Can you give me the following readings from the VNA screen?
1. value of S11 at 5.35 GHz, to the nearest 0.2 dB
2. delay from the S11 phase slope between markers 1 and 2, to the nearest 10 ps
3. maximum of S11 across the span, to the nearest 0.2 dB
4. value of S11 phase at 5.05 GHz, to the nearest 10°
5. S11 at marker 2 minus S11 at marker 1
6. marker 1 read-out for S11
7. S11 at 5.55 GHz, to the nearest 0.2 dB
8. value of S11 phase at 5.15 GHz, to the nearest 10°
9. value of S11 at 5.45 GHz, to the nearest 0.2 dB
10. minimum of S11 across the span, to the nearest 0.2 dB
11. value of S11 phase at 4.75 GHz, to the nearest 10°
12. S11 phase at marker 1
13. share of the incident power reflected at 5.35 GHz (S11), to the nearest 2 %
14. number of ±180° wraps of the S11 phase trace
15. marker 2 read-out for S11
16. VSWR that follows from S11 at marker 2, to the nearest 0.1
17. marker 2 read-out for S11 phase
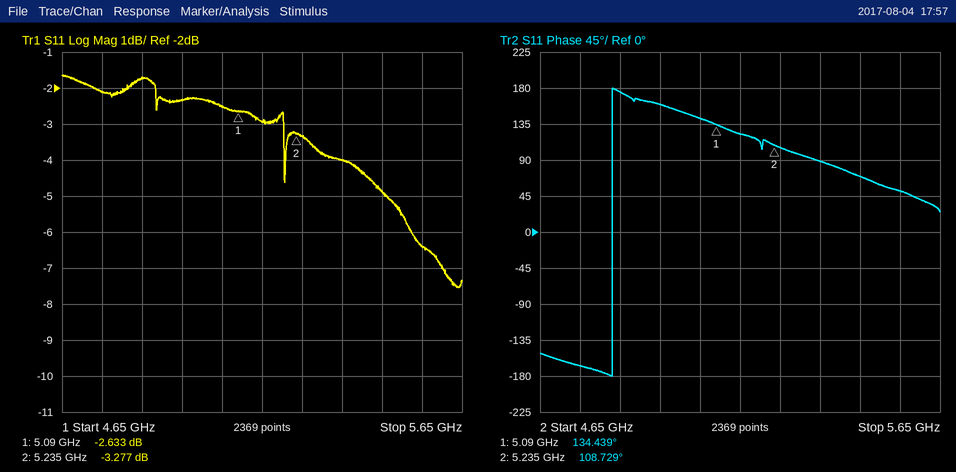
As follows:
-4.0 dB
490 ps
-1.6 dB
140°
-0.644 dB
-2.633 dB
-6.4 dB
120°
-4.8 dB
-7.6 dB
-170°
134.439°
40 %
1
-3.277 dB
5.4
108.729°
